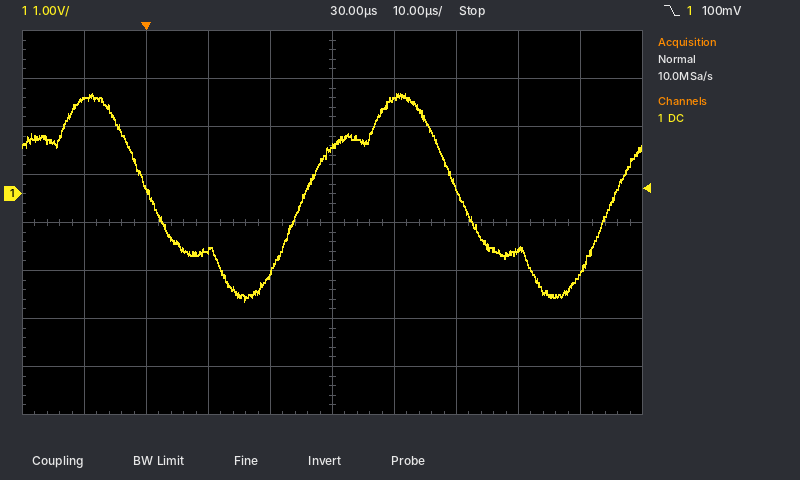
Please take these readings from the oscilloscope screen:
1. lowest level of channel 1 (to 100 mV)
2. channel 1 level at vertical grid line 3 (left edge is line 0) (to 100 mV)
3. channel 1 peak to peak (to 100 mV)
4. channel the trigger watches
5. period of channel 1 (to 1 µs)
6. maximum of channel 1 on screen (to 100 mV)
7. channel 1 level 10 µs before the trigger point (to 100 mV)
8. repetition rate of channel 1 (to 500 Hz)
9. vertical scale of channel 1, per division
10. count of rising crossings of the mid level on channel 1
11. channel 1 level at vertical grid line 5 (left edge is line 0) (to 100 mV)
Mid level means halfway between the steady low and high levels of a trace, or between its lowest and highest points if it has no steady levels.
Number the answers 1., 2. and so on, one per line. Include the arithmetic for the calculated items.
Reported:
1. -2.2 V
2. -1.2 V
3. 2.1 V − (-2.2 V) = 4.3 V
4. channel 1
5. 50 µs
6. 2.1 V
7. 2.0 V
8. 1 / 50 µs ≈ 20.0 kHz
9. 1 V
10. 2
11. 1.0 V
